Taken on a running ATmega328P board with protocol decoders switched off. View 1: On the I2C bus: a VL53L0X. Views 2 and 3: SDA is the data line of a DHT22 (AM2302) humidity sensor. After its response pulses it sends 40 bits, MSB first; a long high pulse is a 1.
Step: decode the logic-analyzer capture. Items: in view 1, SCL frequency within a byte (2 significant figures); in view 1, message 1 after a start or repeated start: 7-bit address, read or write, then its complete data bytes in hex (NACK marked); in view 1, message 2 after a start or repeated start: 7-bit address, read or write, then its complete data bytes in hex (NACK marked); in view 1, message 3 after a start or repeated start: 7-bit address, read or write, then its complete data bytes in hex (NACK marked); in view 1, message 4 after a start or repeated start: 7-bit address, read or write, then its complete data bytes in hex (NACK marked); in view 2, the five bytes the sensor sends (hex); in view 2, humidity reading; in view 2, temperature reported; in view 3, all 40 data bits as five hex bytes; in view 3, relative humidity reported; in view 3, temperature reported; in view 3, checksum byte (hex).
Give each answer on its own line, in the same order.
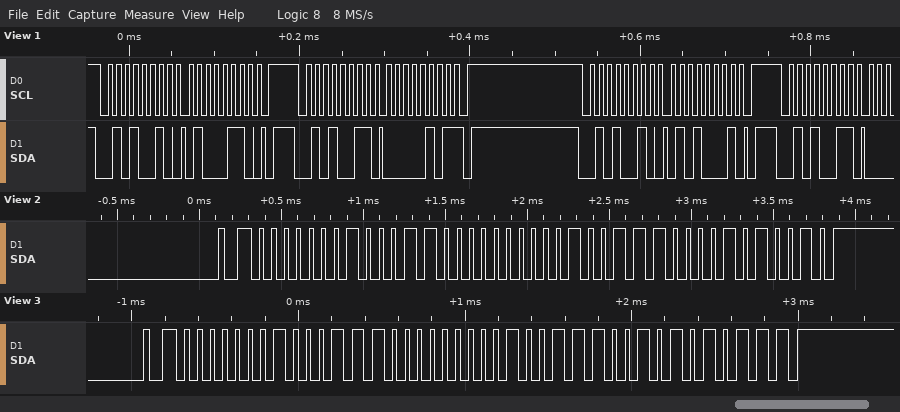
100 kHz
0x29 write: 46
0x29 read: 05 NACK
0x29 write: 51
0x29 read
01 18 01 38 52
28.0 %
31.2 °C
01 1C 01 39 57
28.4 %
31.3 °C
0x57
